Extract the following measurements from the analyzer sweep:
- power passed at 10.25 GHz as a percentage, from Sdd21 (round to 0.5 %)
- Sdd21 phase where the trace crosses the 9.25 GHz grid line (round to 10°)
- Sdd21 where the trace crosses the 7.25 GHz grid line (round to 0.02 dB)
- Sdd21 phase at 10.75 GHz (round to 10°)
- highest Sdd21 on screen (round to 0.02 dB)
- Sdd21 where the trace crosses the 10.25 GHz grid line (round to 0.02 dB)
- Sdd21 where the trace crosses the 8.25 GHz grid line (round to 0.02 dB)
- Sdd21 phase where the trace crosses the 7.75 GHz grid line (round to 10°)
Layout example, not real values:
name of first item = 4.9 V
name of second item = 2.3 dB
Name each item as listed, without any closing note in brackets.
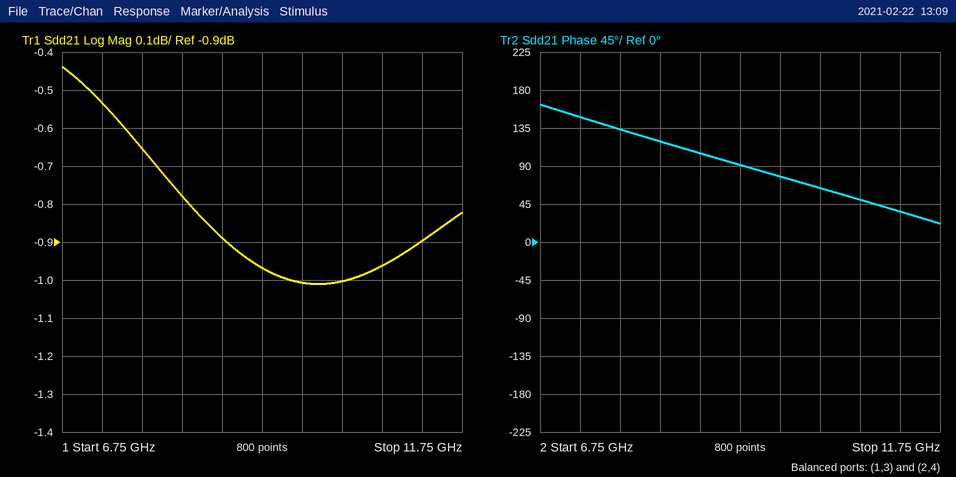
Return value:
power passed at 10.25 GHz as a percentage, from Sdd21 = 79.5 %
Sdd21 phase where the trace crosses the 9.25 GHz grid line = 90°
Sdd21 where the trace crosses the 7.25 GHz grid line = -0.54 dB
Sdd21 phase at 10.75 GHz = 50°
highest Sdd21 on screen = -0.44 dB
Sdd21 where the trace crosses the 10.25 GHz grid line = -1.00 dB
Sdd21 where the trace crosses the 8.25 GHz grid line = -0.78 dB
Sdd21 phase where the trace crosses the 7.75 GHz grid line = 130°
